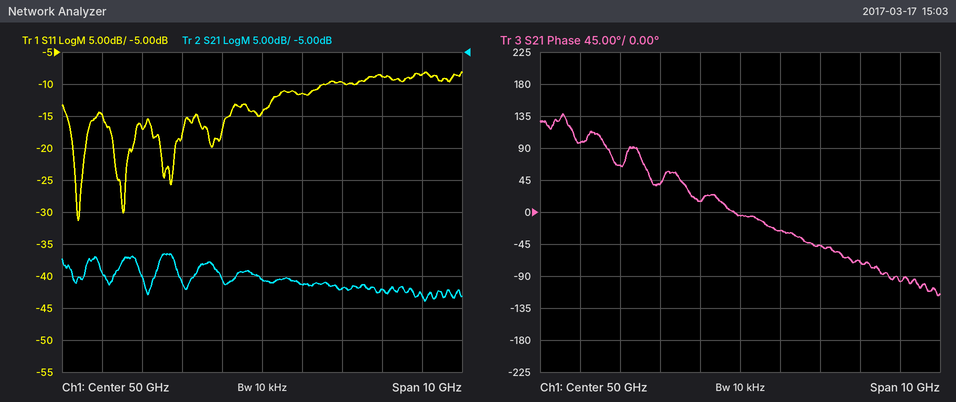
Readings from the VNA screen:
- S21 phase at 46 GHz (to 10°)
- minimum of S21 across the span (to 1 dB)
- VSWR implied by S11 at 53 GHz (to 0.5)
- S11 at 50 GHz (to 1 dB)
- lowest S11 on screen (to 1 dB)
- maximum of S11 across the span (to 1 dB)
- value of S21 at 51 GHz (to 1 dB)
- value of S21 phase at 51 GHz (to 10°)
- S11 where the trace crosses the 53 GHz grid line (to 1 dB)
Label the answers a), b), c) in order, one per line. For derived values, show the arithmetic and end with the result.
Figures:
a) 100°
b) -44 dB
c) |Γ| = 10^(-9/20) = 0.3548; VSWR = (1 + 0.3548)/(1 − 0.3548) ≈ 2.10, so 2.0 to the nearest 0.5
d) -14 dB
e) -31 dB
f) -8 dB
g) -41 dB
h) -30°
i) -9 dB
